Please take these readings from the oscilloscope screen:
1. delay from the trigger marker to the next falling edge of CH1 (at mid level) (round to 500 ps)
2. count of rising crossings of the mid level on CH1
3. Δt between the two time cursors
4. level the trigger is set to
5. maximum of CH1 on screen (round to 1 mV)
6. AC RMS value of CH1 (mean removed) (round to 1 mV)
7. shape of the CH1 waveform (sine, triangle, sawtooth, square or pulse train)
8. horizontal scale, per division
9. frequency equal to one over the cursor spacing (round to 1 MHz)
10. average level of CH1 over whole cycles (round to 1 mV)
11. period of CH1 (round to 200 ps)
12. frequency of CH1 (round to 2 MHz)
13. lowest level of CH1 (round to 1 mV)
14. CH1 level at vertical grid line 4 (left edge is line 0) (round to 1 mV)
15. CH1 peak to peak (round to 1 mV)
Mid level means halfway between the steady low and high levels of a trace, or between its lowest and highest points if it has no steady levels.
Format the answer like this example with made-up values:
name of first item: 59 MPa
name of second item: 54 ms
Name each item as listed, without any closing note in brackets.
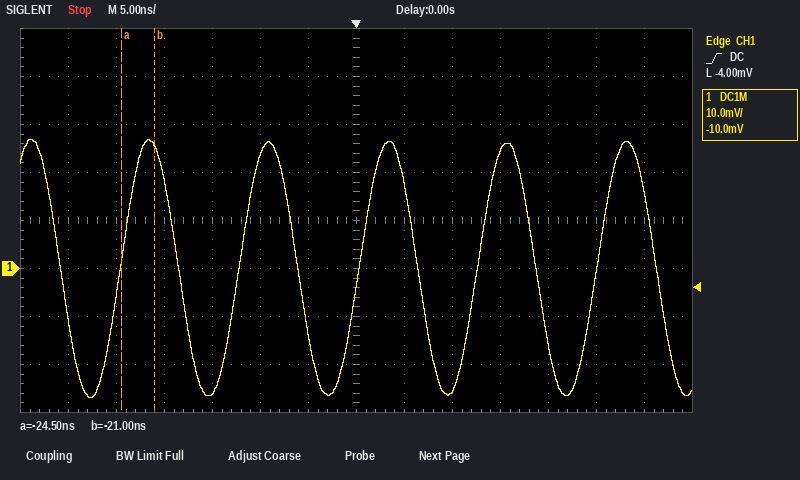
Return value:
delay from the trigger marker to the next falling edge of CH1 (at mid level): 6.5 ns
count of rising crossings of the mid level on CH1: 5
Δt between the two time cursors: 3.5 ns
level the trigger is set to: -4.00 mV
maximum of CH1 on screen: 27 mV
AC RMS value of CH1 (mean removed): 19 mV
shape of the CH1 waveform: sine
horizontal scale, per division: 5 ns
frequency equal to one over the cursor spacing: 286 MHz
average level of CH1 over whole cycles: 0 mV
period of CH1: 12.4 ns
frequency of CH1: 80 MHz
lowest level of CH1: -27 mV
CH1 level at vertical grid line 4 (left edge is line 0): -26 mV
CH1 peak to peak: 54 mV
